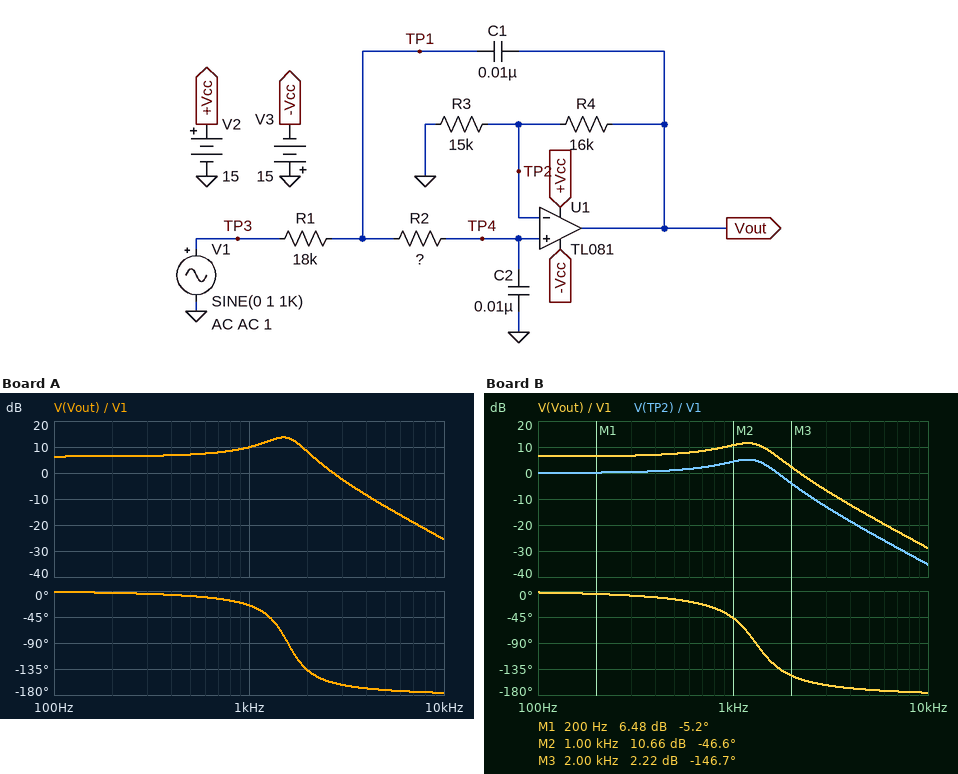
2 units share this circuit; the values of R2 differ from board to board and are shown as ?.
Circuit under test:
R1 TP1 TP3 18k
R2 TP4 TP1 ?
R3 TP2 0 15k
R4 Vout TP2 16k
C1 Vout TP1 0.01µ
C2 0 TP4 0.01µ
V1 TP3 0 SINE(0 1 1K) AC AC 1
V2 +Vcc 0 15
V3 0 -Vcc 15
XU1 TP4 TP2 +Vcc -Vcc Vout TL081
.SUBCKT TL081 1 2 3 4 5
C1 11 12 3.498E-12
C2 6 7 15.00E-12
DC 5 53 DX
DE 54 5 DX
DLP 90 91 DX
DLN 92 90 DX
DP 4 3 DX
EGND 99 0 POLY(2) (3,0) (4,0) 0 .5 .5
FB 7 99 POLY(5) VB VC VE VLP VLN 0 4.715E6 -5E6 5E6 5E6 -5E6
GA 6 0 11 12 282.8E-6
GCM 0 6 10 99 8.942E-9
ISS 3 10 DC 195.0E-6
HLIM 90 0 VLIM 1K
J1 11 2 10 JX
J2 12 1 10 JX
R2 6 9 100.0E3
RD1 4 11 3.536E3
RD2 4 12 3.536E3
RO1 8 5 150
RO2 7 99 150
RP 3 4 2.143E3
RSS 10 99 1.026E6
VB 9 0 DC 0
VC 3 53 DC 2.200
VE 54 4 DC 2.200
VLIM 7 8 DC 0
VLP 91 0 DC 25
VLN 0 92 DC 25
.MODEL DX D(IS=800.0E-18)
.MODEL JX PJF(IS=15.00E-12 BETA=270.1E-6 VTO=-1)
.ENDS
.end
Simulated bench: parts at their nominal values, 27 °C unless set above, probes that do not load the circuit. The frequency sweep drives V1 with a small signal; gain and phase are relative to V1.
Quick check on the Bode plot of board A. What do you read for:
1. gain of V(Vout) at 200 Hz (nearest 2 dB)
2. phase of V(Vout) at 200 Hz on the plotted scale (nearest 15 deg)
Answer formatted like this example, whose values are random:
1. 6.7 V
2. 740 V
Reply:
1. 6 dB
2. 0 deg
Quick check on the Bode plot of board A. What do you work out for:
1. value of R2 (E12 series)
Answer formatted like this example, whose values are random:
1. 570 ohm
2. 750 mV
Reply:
1. 5.6 kΩ
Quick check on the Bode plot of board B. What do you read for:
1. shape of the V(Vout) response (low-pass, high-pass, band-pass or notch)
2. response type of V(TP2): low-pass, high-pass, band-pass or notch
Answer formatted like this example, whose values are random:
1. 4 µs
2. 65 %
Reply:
1. low-pass
2. low-pass
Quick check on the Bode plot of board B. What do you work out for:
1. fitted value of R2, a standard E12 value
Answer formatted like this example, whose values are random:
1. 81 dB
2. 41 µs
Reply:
1. 8.2 kΩ
